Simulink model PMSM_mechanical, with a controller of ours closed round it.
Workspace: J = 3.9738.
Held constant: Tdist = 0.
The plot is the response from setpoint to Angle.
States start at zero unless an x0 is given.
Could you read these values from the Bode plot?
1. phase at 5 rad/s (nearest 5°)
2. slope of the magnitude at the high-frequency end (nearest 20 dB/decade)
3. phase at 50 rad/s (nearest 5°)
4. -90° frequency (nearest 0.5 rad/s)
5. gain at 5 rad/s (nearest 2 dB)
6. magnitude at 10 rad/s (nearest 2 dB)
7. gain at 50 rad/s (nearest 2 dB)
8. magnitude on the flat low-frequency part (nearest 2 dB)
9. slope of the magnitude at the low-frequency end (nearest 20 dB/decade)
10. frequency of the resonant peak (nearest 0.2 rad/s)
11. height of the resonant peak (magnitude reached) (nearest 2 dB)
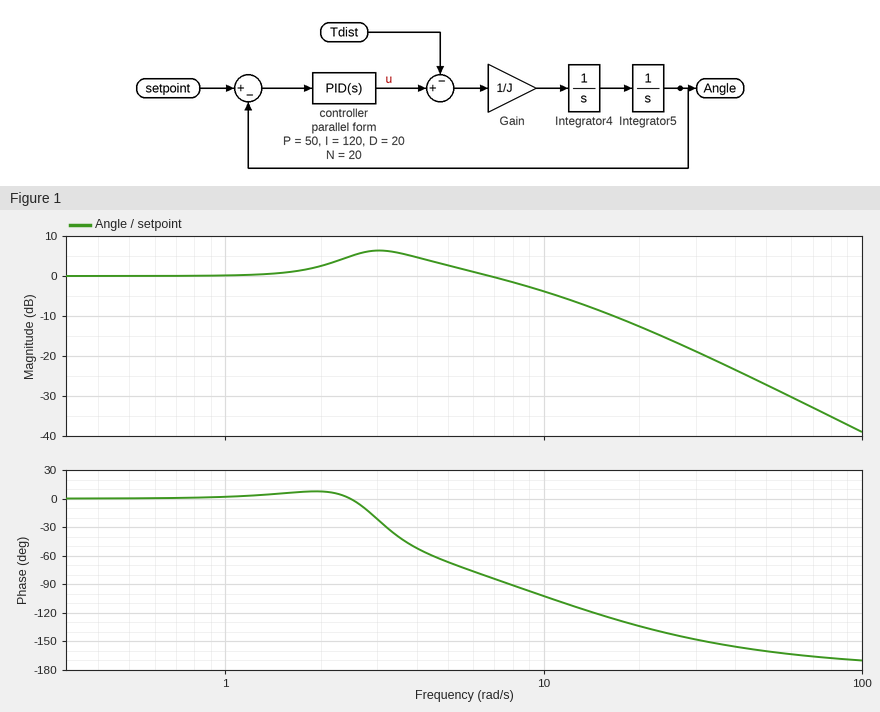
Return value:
-65°
-40 dB/decade
-160°
8.0 rad/s
2 dB
-4 dB
-28 dB
0 dB
0 dB/decade
3.0 rad/s
6 dB
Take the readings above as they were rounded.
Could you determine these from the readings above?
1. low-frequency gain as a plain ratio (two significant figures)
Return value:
1.0
